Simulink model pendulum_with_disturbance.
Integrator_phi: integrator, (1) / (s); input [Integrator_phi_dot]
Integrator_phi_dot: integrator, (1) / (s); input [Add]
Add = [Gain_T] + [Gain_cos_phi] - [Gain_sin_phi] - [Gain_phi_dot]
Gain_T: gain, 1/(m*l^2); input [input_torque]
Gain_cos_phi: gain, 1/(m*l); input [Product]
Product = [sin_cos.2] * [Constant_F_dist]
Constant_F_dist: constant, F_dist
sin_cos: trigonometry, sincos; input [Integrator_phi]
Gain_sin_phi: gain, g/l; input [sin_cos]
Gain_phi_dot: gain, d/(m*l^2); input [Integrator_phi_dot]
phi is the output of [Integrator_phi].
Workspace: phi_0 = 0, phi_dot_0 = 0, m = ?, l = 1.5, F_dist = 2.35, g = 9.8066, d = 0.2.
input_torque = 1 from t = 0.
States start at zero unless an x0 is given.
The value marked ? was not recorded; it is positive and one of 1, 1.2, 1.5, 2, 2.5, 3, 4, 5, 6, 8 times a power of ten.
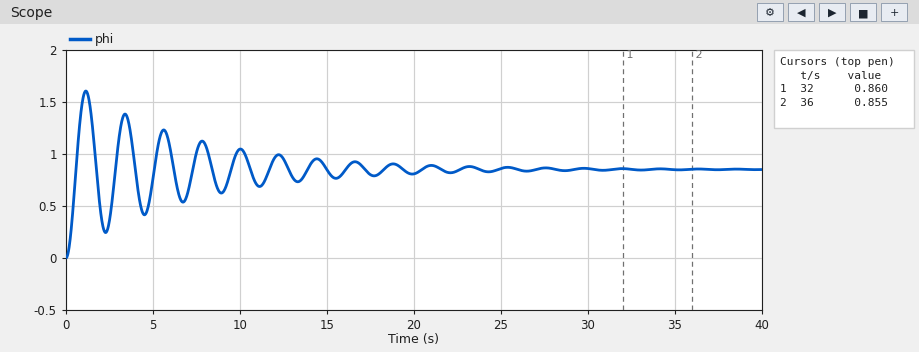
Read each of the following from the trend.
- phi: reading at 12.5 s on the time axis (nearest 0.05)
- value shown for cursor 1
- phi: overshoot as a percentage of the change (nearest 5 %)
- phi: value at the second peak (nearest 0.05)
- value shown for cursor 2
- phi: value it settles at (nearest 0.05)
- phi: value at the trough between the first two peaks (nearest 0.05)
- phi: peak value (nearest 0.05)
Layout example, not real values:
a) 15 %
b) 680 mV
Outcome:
a) 0.95
b) 0.860
c) 90 %
d) 1.40
e) 0.855
f) 0.85
g) 0.25
h) 1.60
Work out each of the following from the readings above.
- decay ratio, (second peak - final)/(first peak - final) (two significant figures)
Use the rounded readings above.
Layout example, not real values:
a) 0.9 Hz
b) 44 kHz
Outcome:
a) 0.73
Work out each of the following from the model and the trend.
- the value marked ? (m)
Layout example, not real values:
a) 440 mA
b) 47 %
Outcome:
a) 0.3
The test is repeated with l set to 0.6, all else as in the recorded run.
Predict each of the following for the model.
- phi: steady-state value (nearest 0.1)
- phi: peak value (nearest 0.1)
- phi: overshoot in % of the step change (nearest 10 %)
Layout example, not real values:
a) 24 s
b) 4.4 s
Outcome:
a) 1.1
b) 1.8
c) 60 %
